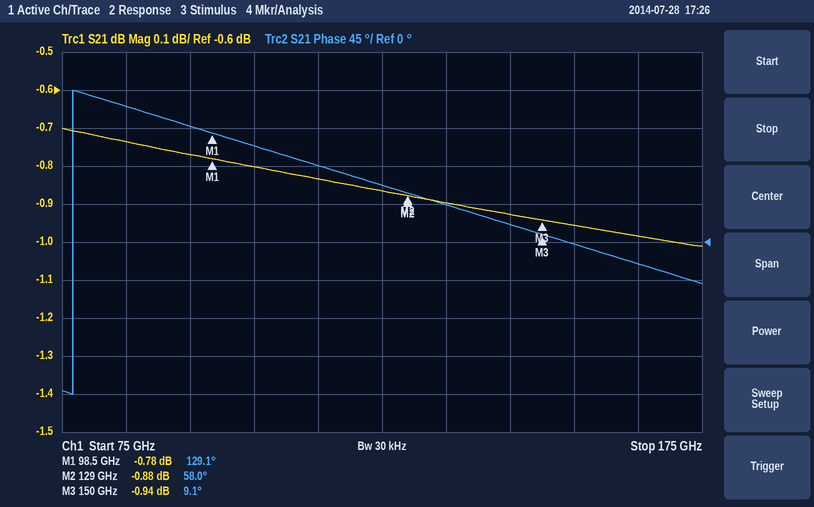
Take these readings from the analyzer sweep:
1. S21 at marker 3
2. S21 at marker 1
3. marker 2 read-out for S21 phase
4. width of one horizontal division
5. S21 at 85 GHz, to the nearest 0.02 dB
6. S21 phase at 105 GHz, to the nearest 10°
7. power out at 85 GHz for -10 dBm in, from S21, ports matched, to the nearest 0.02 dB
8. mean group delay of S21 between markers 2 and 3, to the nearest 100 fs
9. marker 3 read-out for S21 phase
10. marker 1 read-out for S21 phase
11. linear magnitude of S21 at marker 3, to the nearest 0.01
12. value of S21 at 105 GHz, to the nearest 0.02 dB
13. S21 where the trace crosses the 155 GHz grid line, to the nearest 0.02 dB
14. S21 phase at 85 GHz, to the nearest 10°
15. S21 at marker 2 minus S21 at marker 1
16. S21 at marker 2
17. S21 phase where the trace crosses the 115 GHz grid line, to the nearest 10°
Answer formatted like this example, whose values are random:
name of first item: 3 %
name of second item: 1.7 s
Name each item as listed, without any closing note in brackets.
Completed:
S21 at marker 3: -0.94 dB
S21 at marker 1: -0.78 dB
marker 2 read-out for S21 phase: 58.0°
width of one horizontal division: 10 GHz
S21 at 85 GHz, to the nearest 0.02 dB: -0.74 dB
S21 phase at 105 GHz, to the nearest 10°: 110°
power out at 85 GHz for -10 dBm in, from S21, ports matched, to the nearest 0.02 dB: -10.74 dBm
mean group delay of S21 between markers 2 and 3, to the nearest 100 fs: 6.5 ps
marker 3 read-out for S21 phase: 9.1°
marker 1 read-out for S21 phase: 129.1°
linear magnitude of S21 at marker 3, to the nearest 0.01: 0.90
value of S21 at 105 GHz, to the nearest 0.02 dB: -0.80 dB
S21 where the trace crosses the 155 GHz grid line, to the nearest 0.02 dB: -0.96 dB
S21 phase at 85 GHz, to the nearest 10°: 160°
S21 at marker 2 minus S21 at marker 1: -0.10 dB
S21 at marker 2: -0.88 dB
S21 phase where the trace crosses the 115 GHz grid line, to the nearest 10°: 90°
